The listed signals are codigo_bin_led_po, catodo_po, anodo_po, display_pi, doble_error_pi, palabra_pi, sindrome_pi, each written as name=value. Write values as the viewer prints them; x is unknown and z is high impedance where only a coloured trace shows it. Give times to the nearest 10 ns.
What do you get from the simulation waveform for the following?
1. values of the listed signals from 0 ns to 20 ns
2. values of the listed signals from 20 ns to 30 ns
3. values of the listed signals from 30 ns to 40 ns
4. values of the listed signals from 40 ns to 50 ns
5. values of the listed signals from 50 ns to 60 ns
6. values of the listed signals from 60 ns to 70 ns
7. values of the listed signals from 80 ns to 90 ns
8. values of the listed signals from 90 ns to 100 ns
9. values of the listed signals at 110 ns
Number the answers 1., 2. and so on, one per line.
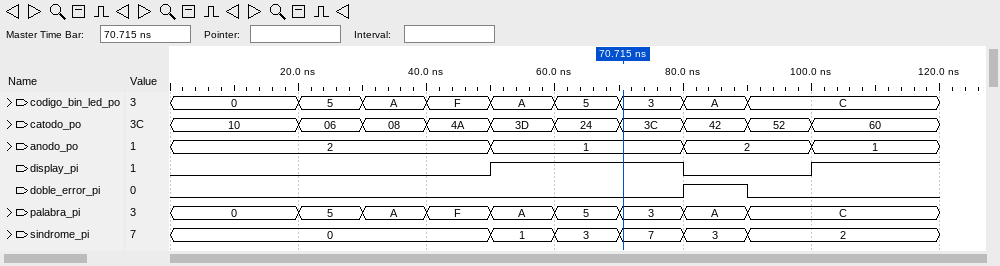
1. codigo_bin_led_po=0, catodo_po=10, anodo_po=2, display_pi=0, doble_error_pi=0, palabra_pi=0, sindrome_pi=0
2. codigo_bin_led_po=5, catodo_po=06, anodo_po=2, display_pi=0, doble_error_pi=0, palabra_pi=5, sindrome_pi=0
3. codigo_bin_led_po=A, catodo_po=08, anodo_po=2, display_pi=0, doble_error_pi=0, palabra_pi=A, sindrome_pi=0
4. codigo_bin_led_po=F, catodo_po=4A, anodo_po=2, display_pi=0, doble_error_pi=0, palabra_pi=F, sindrome_pi=0
5. codigo_bin_led_po=A, catodo_po=3D, anodo_po=1, display_pi=1, doble_error_pi=0, palabra_pi=A, sindrome_pi=1
6. codigo_bin_led_po=5, catodo_po=24, anodo_po=1, display_pi=1, doble_error_pi=0, palabra_pi=5, sindrome_pi=3
7. codigo_bin_led_po=A, catodo_po=42, anodo_po=2, display_pi=0, doble_error_pi=1, palabra_pi=A, sindrome_pi=3
8. codigo_bin_led_po=C, catodo_po=52, anodo_po=2, display_pi=0, doble_error_pi=0, palabra_pi=C, sindrome_pi=2
9. codigo_bin_led_po=C, catodo_po=60, anodo_po=1, display_pi=1, doble_error_pi=0, palabra_pi=C, sindrome_pi=2
